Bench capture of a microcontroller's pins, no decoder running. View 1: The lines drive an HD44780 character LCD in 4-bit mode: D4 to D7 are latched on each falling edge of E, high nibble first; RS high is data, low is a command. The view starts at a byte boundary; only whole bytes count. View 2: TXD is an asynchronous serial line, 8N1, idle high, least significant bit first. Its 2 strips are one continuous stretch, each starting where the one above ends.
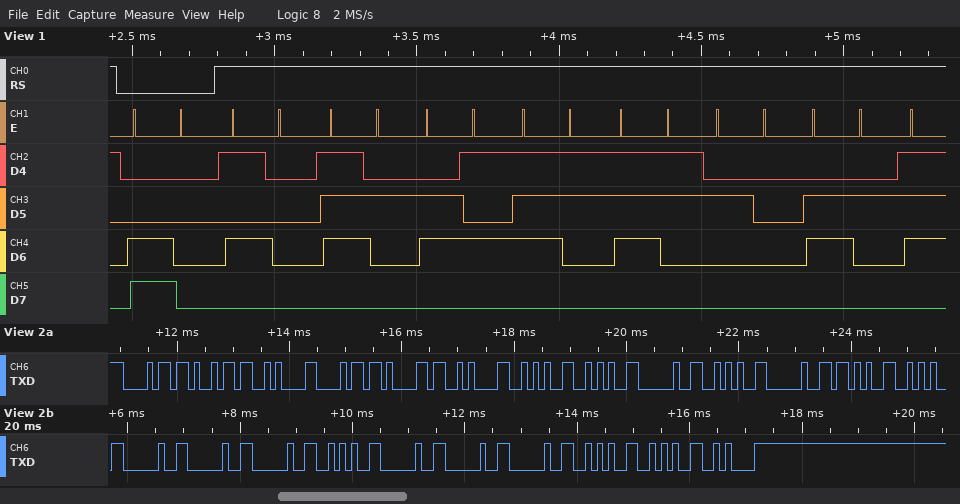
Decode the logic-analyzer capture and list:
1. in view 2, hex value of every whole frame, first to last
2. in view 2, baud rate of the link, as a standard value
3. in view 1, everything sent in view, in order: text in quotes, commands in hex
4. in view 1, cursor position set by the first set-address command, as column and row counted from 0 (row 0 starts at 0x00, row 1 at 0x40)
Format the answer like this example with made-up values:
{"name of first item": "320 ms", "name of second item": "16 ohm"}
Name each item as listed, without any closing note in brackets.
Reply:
{"in view 2, hex value of every whole frame, first to last": "68 69 0A 68 61 0A 2A 2A 20 2A 20 2B 2A 20 20 20 2A 20 20 20 2A 2A 0A", "in view 2, baud rate of the link, as a standard value": "9600 baud", "in view 1, everything sent in view, in order: text in quotes, commands in hex": "0xC0 \"Press b\"", "in view 1, cursor position set by the first set-address command, as column and row counted from 0": "column 0, row 1"}
